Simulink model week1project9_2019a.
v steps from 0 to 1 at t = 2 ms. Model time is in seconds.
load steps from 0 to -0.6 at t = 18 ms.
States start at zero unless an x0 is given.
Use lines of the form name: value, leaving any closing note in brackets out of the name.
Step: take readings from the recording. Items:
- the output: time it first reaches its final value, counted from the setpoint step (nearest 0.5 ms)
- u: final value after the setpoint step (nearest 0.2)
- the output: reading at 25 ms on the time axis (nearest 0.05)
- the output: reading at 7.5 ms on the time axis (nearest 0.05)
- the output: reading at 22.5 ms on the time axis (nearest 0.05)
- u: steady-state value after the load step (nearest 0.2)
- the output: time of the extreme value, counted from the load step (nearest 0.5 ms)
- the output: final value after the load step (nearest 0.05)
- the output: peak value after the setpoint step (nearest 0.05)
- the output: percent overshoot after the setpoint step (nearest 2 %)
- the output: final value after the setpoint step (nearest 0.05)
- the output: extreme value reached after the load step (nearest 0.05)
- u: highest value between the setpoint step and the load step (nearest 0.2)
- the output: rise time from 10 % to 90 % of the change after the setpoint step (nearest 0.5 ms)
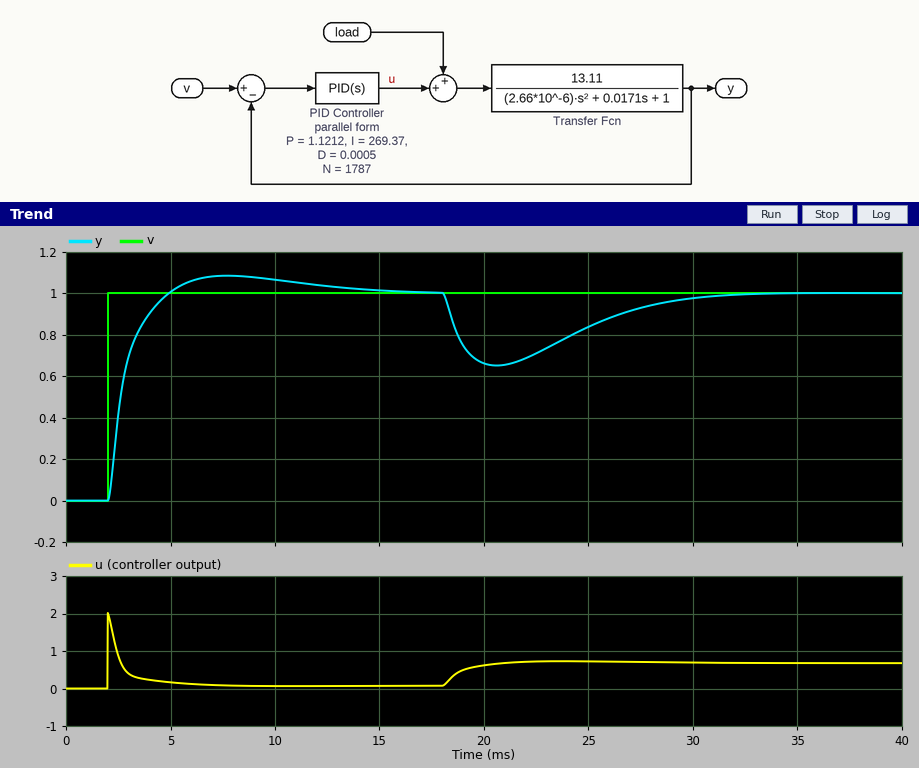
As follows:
the output: time it first reaches its final value, counted from the setpoint step: 3.0 ms
u: final value after the setpoint step: 0.0
the output: reading at 25 ms on the time axis: 0.85
the output: reading at 7.5 ms on the time axis: 1.10
the output: reading at 22.5 ms on the time axis: 0.70
u: steady-state value after the load step: 0.6
the output: time of the extreme value, counted from the load step: 2.5 ms
the output: final value after the load step: 1.00
the output: peak value after the setpoint step: 1.10
the output: percent overshoot after the setpoint step: 8 %
the output: final value after the setpoint step: 1.00
the output: extreme value reached after the load step: 0.65
u: highest value between the setpoint step and the load step: 2.0
the output: rise time from 10 % to 90 % of the change after the setpoint step: 2.0 ms
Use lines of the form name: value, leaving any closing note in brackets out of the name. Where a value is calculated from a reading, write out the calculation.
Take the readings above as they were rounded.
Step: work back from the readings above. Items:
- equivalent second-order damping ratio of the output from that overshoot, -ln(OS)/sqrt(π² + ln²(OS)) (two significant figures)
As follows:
equivalent second-order damping ratio of the output from that overshoot, -ln(OS)/sqrt(π² + ln²(OS)): ln(0.08) = -2.526; 2.526 / sqrt(9.870 + 6.379) = 0.63
